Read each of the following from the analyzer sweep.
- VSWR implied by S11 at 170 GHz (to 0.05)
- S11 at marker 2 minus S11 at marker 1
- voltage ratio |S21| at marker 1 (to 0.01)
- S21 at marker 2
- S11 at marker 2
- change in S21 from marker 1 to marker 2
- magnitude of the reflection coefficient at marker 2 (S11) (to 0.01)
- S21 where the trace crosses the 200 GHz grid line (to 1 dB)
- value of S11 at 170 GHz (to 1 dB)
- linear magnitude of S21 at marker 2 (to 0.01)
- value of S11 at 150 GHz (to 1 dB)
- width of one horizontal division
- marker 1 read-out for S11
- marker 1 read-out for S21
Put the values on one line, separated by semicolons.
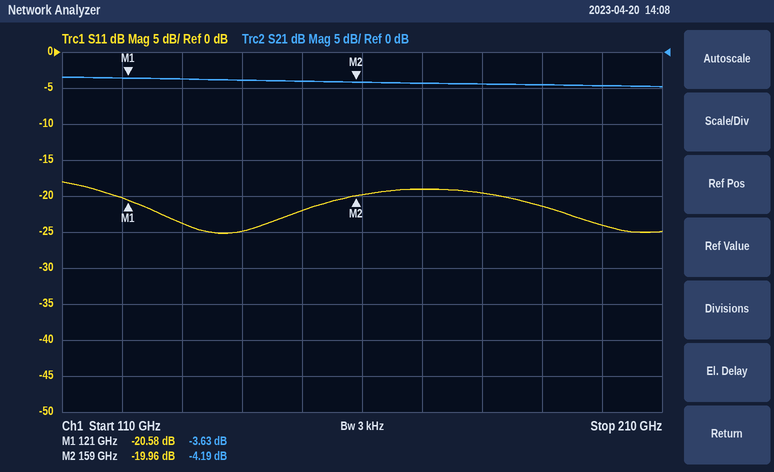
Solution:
1.25; 0.62 dB; 0.66; -4.19 dB; -19.96 dB; -0.56 dB; 0.10; -5 dB; -19 dB; 0.62; -22 dB; 10 GHz; -20.58 dB; -3.63 dB
